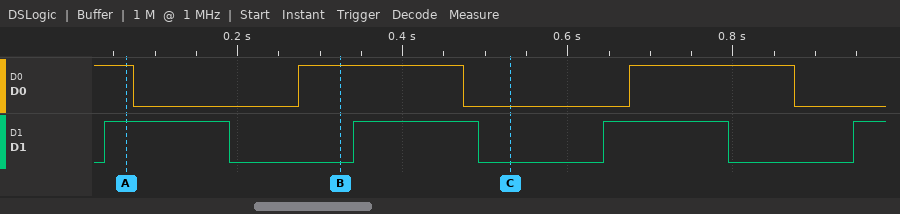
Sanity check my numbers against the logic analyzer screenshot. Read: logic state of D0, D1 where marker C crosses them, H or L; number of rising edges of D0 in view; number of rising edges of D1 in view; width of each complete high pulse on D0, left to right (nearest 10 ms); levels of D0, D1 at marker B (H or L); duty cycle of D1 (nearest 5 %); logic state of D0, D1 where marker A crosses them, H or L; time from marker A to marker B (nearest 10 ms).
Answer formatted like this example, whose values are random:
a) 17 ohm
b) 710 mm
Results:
a) D0=L, D1=L
b) 2
c) 4
d) 200 ms, 200 ms
e) D0=H, D1=L
f) 50 %
g) D0=H, D1=H
h) 260 ms
